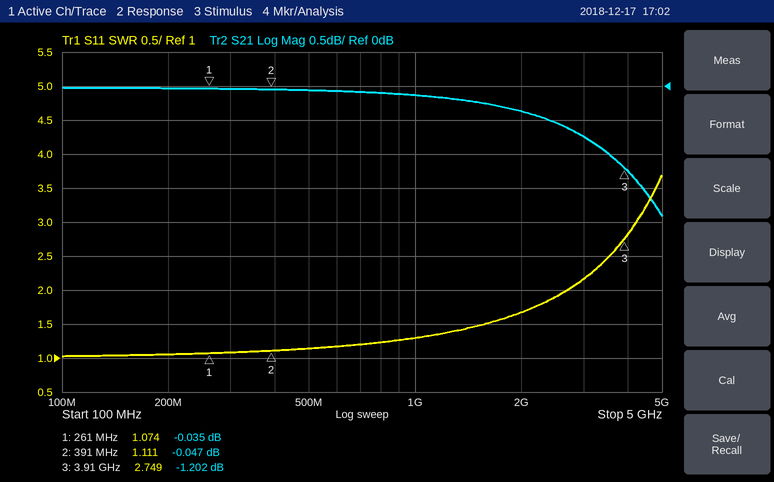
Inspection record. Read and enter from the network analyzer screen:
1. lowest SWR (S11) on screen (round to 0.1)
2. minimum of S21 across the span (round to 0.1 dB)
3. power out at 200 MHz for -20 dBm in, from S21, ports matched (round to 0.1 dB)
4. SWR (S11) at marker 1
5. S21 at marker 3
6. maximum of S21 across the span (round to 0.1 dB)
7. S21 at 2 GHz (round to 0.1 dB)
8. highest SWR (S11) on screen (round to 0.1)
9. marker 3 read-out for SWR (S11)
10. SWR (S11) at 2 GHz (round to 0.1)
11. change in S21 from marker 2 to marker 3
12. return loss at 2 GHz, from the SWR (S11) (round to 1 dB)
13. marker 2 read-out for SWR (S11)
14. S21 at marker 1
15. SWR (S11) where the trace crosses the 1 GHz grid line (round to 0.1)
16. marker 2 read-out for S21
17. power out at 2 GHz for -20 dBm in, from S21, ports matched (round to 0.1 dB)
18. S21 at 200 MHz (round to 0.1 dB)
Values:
1.0
-1.9 dB
-20.0 dBm
1.074
-1.202 dB
0.0 dB
-0.4 dB
3.7
2.749
1.7
-1.155 dB
12 dB
1.111
-0.035 dB
1.3
-0.047 dB
-20.4 dBm
0.0 dB
